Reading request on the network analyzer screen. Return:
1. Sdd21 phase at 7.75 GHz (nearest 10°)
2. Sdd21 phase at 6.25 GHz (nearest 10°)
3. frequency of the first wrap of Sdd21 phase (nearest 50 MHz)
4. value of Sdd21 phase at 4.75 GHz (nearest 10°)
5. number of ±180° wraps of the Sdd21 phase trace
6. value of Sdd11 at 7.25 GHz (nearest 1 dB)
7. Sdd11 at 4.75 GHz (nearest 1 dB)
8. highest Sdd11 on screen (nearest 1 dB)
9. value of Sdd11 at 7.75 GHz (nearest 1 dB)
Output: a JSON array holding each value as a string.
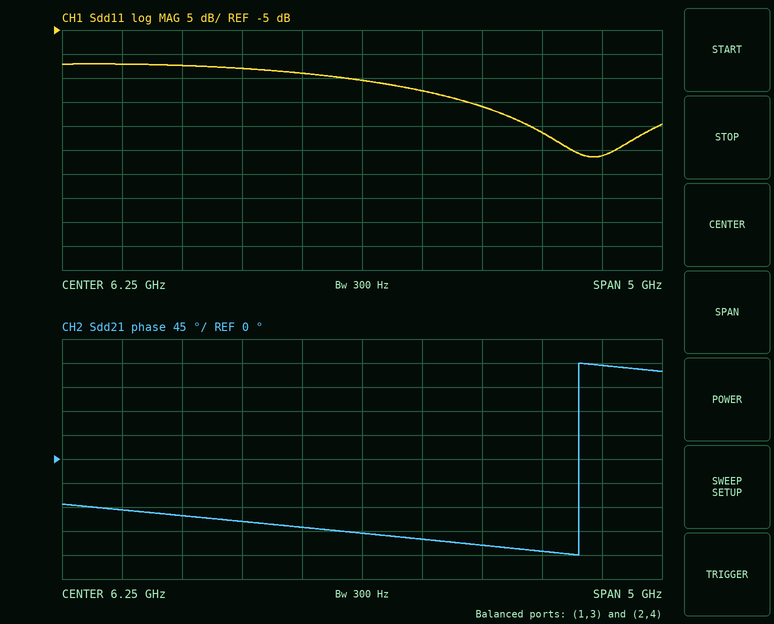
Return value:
["-170°", "-140°", "8.05 GHz", "-110°", "1", "-21 dB", "-12 dB", "-12 dB", "-26 dB"]
